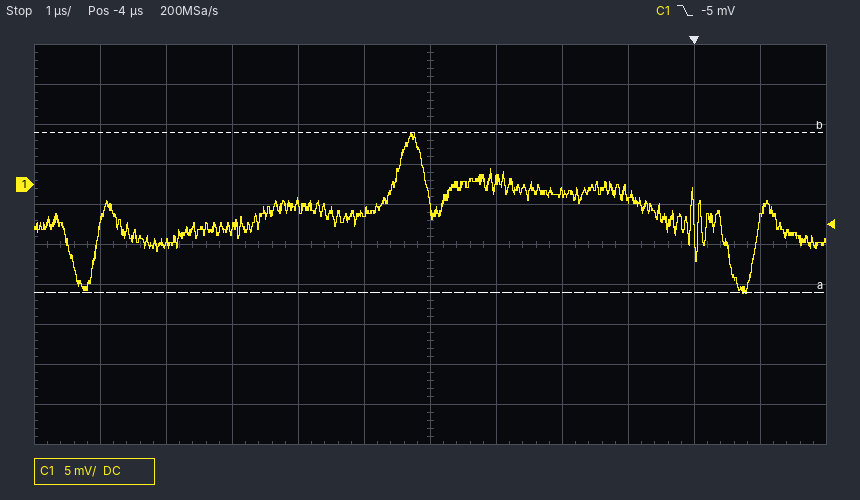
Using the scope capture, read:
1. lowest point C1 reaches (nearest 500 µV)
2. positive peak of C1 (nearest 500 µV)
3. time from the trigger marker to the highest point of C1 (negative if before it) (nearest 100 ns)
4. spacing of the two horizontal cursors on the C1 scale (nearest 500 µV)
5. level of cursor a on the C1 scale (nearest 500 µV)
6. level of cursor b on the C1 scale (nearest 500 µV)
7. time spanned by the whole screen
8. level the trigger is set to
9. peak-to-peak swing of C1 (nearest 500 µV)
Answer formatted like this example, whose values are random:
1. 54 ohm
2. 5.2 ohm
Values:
1. -13.5 mV
2. 6.5 mV
3. -4.3 µs
4. 20.0 mV
5. -13.5 mV
6. 6.5 mV
7. 12 µs
8. -5 mV
9. 20.0 mV
